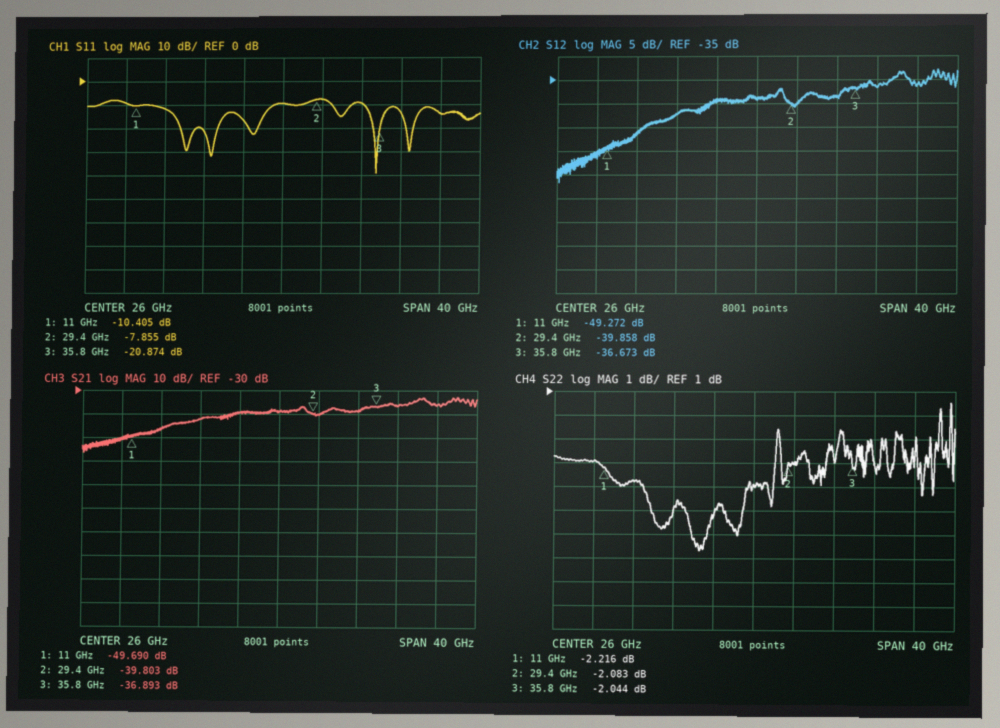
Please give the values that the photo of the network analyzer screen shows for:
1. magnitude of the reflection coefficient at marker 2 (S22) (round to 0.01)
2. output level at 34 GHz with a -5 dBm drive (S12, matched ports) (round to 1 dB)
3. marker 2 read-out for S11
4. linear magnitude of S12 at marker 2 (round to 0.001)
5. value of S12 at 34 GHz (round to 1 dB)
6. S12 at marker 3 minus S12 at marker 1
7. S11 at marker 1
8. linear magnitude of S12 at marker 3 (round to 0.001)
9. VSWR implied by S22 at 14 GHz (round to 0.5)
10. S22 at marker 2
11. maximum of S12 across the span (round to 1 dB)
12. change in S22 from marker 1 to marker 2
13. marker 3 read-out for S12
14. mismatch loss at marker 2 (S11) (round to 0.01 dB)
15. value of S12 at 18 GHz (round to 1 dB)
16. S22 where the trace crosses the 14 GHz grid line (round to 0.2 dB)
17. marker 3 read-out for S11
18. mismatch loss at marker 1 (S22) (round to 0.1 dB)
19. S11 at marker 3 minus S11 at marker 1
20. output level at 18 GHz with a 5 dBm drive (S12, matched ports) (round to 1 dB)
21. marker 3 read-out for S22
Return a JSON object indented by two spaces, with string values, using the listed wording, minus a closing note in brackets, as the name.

{
  "magnitude of the reflection coefficient at marker 2 (S22)": "0.79",
  "output level at 34 GHz with a -5 dBm drive (S12, matched ports)": "-44 dBm",
  "marker 2 read-out for S11": "-7.855 dB",
  "linear magnitude of S12 at marker 2": "0.010",
  "value of S12 at 34 GHz": "-39 dB",
  "S12 at marker 3 minus S12 at marker 1": "12.599 dB",
  "S11 at marker 1": "-10.405 dB",
  "linear magnitude of S12 at marker 3": "0.015",
  "VSWR implied by S22 at 14 GHz": "6.5",
  "S22 at marker 2": "-2.083 dB",
  "maximum of S12 across the span": "-33 dB",
  "change in S22 from marker 1 to marker 2": "0.133 dB",
  "marker 3 read-out for S12": "-36.673 dB",
  "mismatch loss at marker 2 (S11)": "0.78 dB",
  "value of S12 at 18 GHz": "-42 dB",
  "S22 where the trace crosses the 14 GHz grid line": "-2.8 dB",
  "marker 3 read-out for S11": "-20.874 dB",
  "mismatch loss at marker 1 (S22)": "4.0 dB",
  "S11 at marker 3 minus S11 at marker 1": "-10.469 dB",
  "output level at 18 GHz with a 5 dBm drive (S12, matched ports)": "-37 dBm",
  "marker 3 read-out for S22": "-2.044 dB"
}
